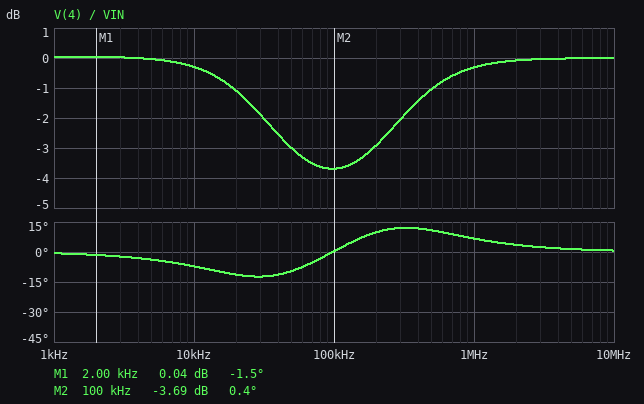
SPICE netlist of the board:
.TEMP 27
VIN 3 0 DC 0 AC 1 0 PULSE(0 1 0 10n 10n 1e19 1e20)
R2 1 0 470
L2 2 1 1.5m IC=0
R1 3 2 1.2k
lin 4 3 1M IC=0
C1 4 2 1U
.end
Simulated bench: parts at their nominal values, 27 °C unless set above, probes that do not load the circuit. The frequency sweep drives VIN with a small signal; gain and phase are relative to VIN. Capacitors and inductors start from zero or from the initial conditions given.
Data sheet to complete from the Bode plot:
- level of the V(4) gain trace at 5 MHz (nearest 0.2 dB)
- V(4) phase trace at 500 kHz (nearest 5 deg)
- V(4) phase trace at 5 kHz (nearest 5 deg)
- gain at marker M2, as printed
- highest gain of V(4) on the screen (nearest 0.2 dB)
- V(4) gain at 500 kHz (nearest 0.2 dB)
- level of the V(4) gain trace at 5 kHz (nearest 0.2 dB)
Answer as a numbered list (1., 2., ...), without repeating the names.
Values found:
1. 0 dB
2. 10 deg
3. -5 deg
4. -3.69 dB
5. 0 dB
6. -1.0 dB
7. 0 dB
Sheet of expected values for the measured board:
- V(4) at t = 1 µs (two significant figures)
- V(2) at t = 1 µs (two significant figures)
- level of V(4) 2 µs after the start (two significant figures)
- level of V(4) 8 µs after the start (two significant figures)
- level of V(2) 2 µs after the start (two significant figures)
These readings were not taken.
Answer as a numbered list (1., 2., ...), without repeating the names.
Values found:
1. 710 mV
2. 710 mV
3. 720 mV
4. 900 mV
5. 720 mV
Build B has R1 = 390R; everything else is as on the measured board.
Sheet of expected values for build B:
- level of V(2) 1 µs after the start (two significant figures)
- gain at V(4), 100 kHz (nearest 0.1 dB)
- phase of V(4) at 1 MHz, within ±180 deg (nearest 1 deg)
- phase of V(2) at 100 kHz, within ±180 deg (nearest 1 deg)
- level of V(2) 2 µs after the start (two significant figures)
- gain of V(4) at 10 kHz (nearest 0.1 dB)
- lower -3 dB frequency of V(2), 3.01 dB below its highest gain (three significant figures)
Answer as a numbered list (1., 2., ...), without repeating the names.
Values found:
1. 840 mV
2. -2.1 dB
3. 2 deg
4. 7 deg
5. 790 mV
6. -0.4 dB
7. 468 Hz
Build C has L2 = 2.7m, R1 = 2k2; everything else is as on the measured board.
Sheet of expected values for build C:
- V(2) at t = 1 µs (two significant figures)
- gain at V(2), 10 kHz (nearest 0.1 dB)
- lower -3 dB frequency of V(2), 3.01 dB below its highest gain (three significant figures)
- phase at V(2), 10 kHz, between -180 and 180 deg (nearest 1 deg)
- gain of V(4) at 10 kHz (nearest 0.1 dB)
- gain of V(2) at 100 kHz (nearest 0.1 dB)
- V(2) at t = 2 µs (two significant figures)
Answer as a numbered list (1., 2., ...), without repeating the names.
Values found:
1. 770 mV
2. -0.3 dB
3. 394 Hz
4. -5 deg
5. -0.4 dB
6. -2.6 dB
7. 780 mV
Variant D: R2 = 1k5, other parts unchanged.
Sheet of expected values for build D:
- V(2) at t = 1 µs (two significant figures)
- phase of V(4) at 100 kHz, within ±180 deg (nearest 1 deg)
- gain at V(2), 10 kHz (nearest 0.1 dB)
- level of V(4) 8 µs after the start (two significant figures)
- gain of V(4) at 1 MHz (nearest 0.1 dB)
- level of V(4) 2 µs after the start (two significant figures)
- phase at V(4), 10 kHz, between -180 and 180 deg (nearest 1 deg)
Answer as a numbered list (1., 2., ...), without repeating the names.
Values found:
1. 790 mV
2. -7 deg
3. 0 dB
4. 990 mV
5. -0.4 dB
6. 850 mV
7. -2 deg
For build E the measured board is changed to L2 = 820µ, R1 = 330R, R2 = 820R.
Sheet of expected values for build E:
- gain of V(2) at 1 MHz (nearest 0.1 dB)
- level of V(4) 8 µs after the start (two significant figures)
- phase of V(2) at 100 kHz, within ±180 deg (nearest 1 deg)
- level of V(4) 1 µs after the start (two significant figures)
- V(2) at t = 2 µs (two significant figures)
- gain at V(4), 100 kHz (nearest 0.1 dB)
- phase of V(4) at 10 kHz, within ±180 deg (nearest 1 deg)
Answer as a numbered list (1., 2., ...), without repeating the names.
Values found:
1. -0.1 dB
2. 950 mV
3. 1 deg
4. 820 mV
5. 810 mV
6. -2.3 dB
7. -4 deg
